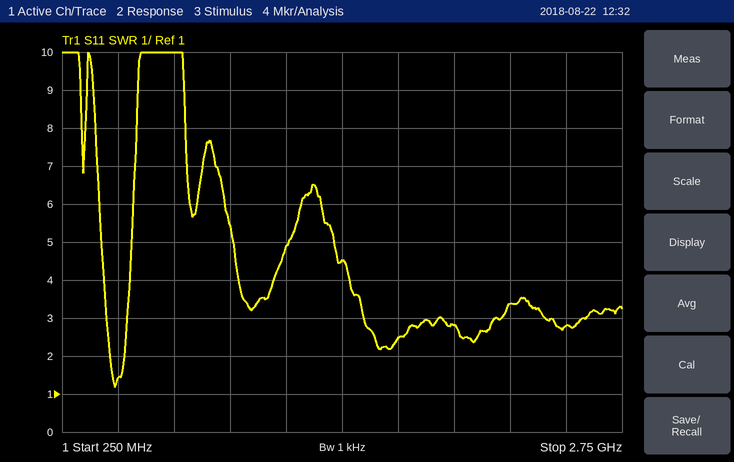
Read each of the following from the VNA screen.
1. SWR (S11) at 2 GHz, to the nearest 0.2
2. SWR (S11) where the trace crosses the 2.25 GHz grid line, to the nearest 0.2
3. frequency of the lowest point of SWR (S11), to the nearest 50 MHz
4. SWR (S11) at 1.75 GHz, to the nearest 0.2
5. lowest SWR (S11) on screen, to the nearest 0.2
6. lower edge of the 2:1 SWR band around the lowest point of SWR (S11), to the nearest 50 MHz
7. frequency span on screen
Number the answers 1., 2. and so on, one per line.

1. 2.8
2. 3.4
3. 500 MHz
4. 2.4
5. 1.2
6. 450 MHz
7. 2.5 GHz
